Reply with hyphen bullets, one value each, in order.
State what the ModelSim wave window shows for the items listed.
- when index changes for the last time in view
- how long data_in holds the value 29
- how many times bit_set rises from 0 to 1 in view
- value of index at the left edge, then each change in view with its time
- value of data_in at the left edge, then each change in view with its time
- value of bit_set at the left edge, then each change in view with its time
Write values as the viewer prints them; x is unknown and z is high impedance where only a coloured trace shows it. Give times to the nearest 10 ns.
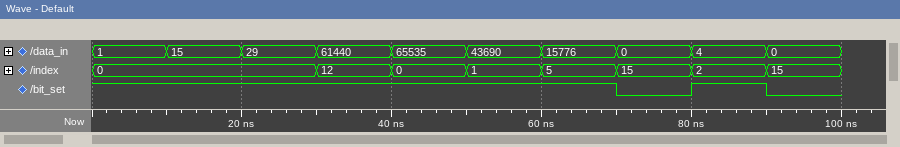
- 90 ns
- 10 ns
- 1
- 0, 12 at 30 ns, 0 at 40 ns, 1 at 50 ns, 5 at 60 ns, 15 at 70 ns, 2 at 80 ns, 15 at 90 ns
- 1, 15 at 10 ns, 29 at 20 ns, 61440 at 30 ns, 65535 at 40 ns, 43690 at 50 ns, 15776 at 60 ns, 0 at 70 ns, 4 at 80 ns, 0 at 90 ns
- 1, 0 at 70 ns, 1 at 80 ns, 0 at 90 ns
